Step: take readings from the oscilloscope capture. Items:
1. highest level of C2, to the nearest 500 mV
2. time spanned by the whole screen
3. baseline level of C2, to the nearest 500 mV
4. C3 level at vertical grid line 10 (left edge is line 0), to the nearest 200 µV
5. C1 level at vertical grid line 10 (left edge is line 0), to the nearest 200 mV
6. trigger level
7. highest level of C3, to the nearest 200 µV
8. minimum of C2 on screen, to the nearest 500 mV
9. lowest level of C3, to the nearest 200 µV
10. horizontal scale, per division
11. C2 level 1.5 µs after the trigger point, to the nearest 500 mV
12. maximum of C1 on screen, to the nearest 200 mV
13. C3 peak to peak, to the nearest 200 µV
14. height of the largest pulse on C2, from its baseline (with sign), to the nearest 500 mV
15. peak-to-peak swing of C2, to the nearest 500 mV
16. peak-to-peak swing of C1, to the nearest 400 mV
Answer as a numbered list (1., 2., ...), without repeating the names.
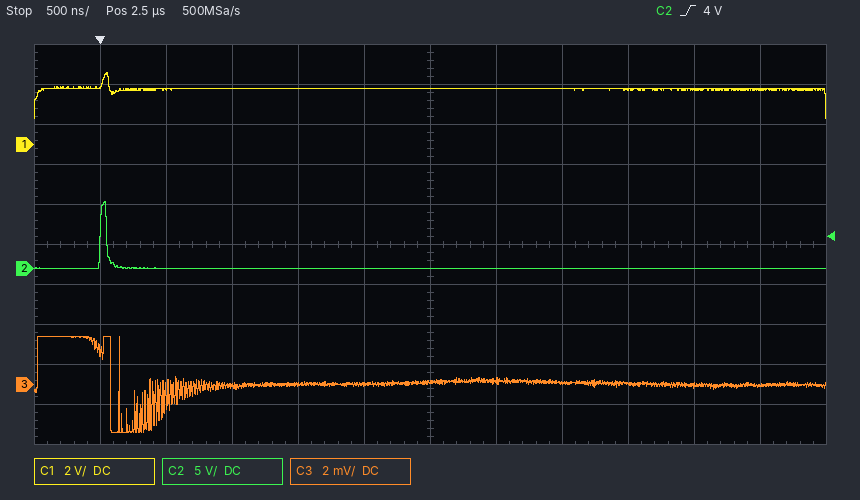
1. 8.5 V
2. 6 µs
3. 0.0 V
4. 0.0 mV
5. 2.8 V
6. 4 V
7. 2.4 mV
8. 0.0 V
9. -2.4 mV
10. 500 ns
11. 0.0 V
12. 3.6 V
13. 4.8 mV
14. +8.5 V
15. 8.5 V
16. 2.4 V
